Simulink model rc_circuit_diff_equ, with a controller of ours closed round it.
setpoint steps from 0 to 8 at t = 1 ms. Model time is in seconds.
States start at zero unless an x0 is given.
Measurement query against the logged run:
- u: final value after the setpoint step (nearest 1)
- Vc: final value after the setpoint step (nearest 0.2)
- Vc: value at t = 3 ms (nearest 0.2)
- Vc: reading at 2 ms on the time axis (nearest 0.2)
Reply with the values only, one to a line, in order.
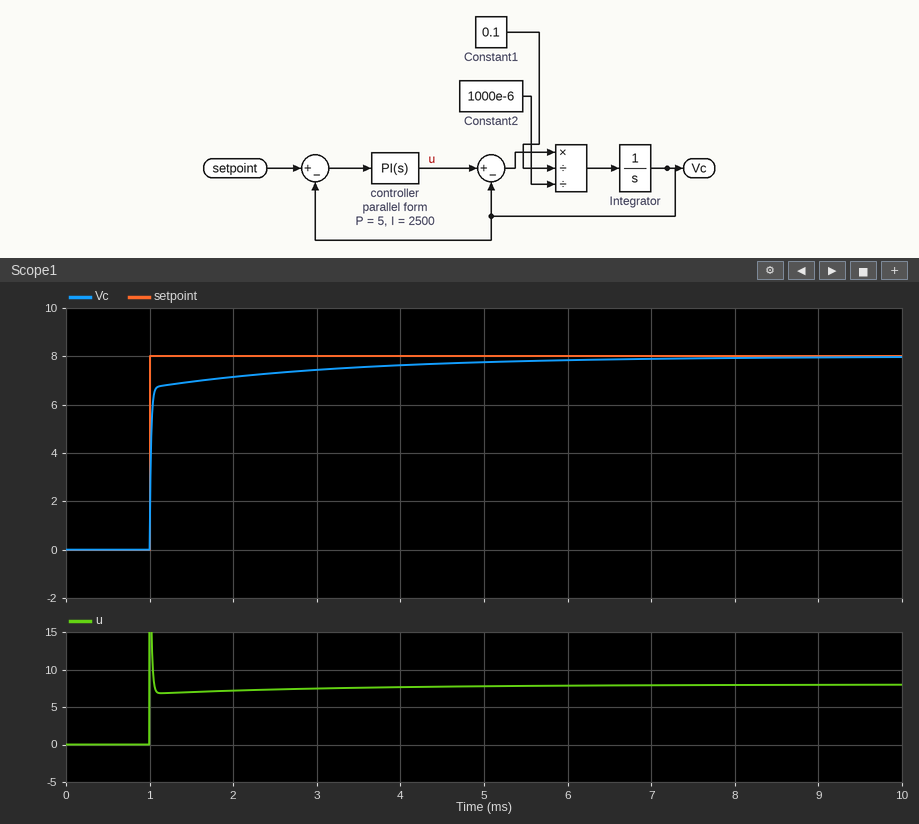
8
8.0
7.4
7.2
